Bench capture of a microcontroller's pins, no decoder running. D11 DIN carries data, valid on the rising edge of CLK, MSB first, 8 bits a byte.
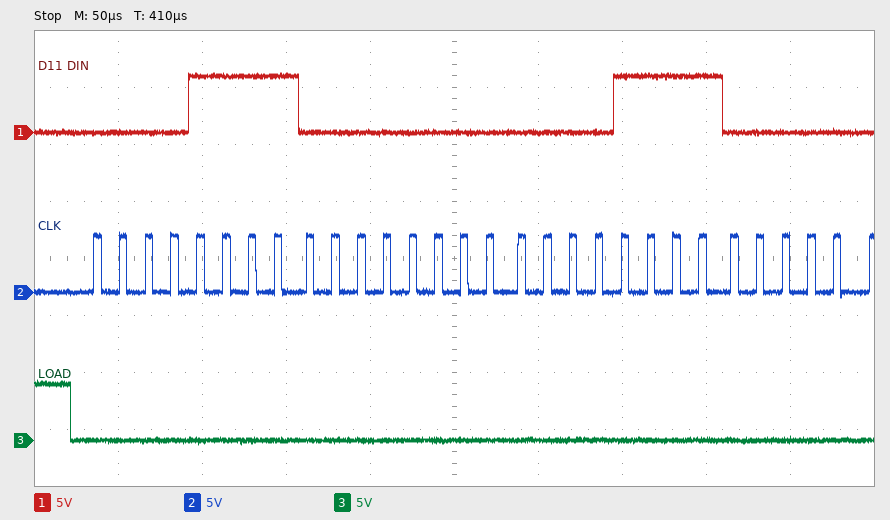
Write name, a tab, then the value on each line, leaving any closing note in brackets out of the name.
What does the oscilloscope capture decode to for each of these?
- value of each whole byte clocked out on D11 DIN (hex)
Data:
value of each whole byte clocked out on D11 DIN	0F 00 0F
